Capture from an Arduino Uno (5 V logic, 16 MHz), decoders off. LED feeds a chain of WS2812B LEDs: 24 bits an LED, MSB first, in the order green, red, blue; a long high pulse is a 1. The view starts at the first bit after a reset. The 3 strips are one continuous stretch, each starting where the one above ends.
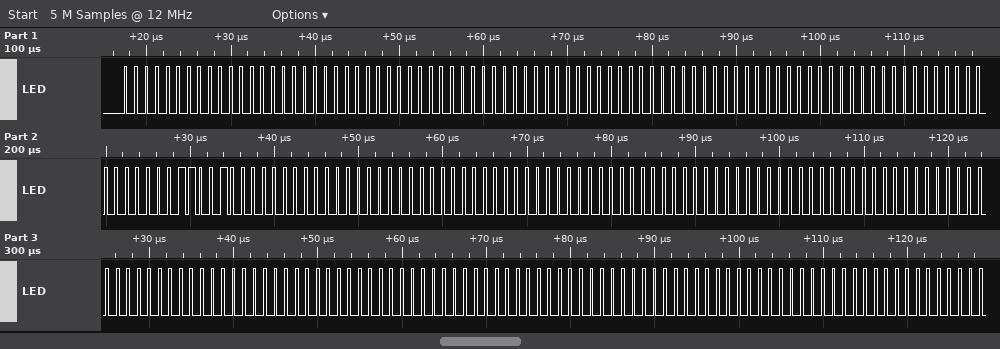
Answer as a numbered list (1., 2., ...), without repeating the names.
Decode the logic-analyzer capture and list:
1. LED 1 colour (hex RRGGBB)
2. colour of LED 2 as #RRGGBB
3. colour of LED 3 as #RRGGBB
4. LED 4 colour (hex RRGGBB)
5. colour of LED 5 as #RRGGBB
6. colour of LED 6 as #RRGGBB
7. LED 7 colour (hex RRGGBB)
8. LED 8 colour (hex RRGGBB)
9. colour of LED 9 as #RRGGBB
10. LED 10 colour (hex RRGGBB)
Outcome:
1. #000000
2. #000000
3. #000000
4. #000064
5. #000000
6. #000000
7. #000000
8. #000000
9. #000000
10. #000000
